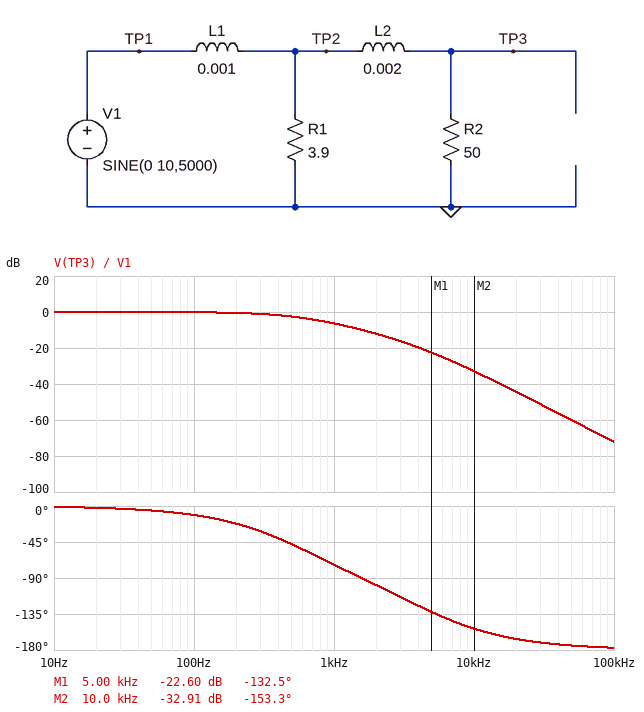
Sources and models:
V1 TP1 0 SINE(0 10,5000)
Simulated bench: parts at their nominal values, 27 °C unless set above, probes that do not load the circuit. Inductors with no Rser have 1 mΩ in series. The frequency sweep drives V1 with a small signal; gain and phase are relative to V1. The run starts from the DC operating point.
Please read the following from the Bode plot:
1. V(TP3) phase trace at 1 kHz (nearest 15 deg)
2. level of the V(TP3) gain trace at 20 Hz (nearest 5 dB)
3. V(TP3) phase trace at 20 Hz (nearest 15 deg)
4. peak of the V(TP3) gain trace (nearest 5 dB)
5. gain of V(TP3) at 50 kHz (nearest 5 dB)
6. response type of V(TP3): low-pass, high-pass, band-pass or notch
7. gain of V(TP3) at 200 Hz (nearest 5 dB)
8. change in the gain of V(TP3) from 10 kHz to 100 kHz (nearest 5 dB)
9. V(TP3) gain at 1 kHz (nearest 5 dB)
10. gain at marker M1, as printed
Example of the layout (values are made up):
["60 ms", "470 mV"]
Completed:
["-75 deg", "0 dB", "0 deg", "0 dB", "-60 dB", "low-pass", "0 dB", "-40 dB", "-5 dB", "-22.60 dB"]
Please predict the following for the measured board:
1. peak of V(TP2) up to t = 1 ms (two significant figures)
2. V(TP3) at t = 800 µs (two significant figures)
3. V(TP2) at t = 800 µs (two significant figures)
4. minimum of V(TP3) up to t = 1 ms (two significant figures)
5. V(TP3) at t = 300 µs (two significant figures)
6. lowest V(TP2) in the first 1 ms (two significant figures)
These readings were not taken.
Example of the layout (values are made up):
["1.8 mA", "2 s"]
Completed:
["2.0 V", "-470 mV", "-1.1 V", "-670 mV", "990 mV", "-1.2 V"]
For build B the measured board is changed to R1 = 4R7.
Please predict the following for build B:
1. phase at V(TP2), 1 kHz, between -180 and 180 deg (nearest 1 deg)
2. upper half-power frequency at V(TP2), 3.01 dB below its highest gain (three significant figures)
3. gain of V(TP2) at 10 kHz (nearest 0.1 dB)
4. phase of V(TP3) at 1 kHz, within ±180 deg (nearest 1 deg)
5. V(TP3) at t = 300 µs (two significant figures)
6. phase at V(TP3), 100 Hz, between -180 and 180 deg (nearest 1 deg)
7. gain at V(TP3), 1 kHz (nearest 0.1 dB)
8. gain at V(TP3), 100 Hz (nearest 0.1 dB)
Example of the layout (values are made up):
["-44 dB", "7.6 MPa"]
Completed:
["-55 deg", "676 Hz", "-22.7 dB", "-69 deg", "1.1 V", "-10 deg", "-5.3 dB", "-0.1 dB"]
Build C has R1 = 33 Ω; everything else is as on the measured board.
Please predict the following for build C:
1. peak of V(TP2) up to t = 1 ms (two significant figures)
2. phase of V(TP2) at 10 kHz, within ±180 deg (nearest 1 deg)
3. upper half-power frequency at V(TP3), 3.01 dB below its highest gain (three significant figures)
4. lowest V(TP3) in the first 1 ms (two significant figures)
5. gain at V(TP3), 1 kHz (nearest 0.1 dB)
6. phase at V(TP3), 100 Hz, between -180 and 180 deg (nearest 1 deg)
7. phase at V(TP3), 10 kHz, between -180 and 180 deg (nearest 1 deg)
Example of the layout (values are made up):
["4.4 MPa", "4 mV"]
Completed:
["6.5 V", "-55 deg", "2.06 kHz", "-3.5 V", "-0.9 dB", "-3 deg", "-124 deg"]
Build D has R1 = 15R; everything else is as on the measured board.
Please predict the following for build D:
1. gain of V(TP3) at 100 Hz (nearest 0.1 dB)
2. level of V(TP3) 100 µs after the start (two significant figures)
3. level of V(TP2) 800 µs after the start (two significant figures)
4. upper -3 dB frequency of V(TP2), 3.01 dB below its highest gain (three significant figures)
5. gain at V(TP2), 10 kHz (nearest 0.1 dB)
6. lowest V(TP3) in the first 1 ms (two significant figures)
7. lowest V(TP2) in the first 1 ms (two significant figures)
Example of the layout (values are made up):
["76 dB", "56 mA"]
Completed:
["0 dB", "3.6 V", "-3.3 V", "1.74 kHz", "-13.2 dB", "-2.3 V", "-3.7 V"]
